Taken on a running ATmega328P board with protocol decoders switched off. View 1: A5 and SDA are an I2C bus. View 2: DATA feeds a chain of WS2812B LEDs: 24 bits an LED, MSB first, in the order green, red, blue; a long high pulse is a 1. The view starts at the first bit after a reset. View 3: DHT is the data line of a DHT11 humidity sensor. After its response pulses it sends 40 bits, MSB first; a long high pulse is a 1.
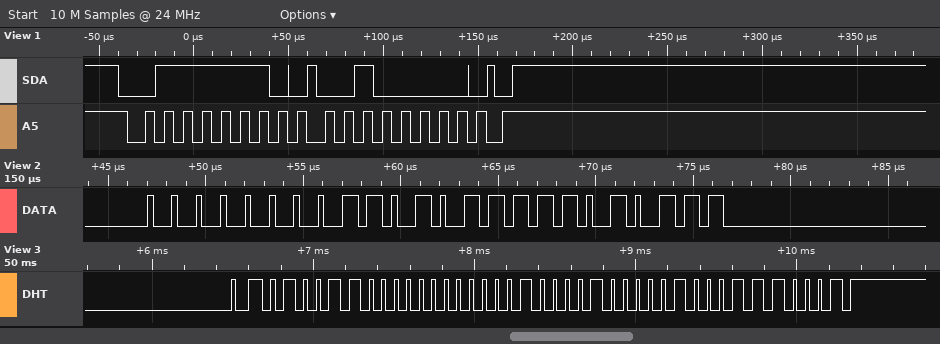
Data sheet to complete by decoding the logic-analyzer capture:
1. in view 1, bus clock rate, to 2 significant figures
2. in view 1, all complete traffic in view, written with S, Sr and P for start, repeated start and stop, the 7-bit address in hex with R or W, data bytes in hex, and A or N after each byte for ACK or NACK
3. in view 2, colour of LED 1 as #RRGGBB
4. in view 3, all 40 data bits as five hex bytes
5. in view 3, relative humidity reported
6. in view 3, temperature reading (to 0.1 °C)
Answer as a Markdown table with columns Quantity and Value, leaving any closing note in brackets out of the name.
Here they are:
| Quantity | Value |
|---|---|
| in view 1, bus clock rate, to 2 significant figures | 100 kHz |
| in view 1, all complete traffic in view, written with S, Sr and P for start, repeated start and stop, the 7-bit address in hex with R or W, data bytes in hex, and A or N after each byte for ACK or NACK | S 3FW A 20 A P |
| in view 2, colour of LED 1 as #RRGGBB | #D700D7 |
| in view 3, all 40 data bits as five hex bytes | 4C 00 21 04 71 |
| in view 3, relative humidity reported | 76 % |
| in view 3, temperature reading | 33.4 °C |
